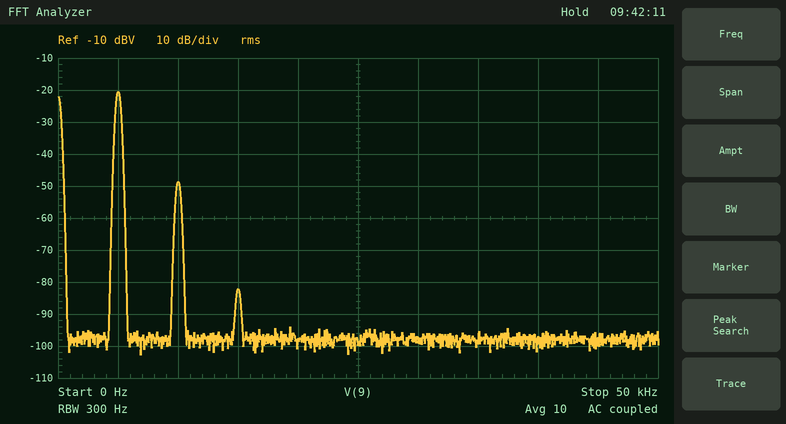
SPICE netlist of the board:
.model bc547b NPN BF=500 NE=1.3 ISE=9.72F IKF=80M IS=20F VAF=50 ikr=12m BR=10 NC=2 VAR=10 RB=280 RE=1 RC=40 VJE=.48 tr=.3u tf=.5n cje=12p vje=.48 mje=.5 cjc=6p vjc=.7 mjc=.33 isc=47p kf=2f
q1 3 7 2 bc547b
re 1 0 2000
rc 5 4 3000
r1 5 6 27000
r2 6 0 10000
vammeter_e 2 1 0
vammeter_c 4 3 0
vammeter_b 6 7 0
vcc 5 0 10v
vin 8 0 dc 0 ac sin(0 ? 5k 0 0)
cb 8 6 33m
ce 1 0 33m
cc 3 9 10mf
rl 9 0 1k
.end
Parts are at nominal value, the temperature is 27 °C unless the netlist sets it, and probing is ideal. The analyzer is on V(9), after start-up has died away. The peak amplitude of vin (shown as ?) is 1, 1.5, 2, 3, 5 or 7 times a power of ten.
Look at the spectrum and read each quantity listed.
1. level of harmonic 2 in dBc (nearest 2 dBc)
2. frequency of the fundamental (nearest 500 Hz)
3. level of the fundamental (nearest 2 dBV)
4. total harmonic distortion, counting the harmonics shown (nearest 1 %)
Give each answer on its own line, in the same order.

-28 dBc
5.0 kHz
-20 dBV
4 %
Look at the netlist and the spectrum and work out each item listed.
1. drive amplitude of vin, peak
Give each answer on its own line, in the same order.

5 mV
